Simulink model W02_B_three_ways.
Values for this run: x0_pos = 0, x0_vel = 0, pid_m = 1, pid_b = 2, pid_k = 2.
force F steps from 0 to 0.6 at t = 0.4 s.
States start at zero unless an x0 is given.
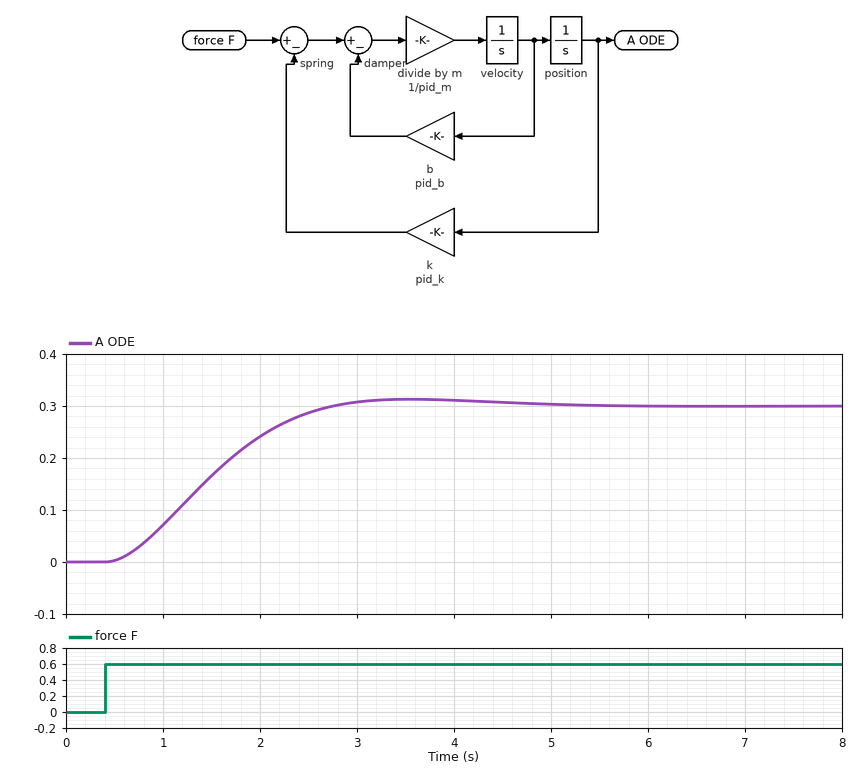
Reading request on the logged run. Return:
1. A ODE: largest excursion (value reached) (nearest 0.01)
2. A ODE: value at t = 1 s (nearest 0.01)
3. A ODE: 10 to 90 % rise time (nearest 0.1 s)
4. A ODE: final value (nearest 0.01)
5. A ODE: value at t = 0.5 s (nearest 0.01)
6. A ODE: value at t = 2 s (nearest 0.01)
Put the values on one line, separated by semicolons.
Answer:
0.31; 0.07; 1.5 s; 0.30; 0.00; 0.24
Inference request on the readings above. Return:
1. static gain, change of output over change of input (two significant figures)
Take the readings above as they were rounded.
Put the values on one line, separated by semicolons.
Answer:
0.50
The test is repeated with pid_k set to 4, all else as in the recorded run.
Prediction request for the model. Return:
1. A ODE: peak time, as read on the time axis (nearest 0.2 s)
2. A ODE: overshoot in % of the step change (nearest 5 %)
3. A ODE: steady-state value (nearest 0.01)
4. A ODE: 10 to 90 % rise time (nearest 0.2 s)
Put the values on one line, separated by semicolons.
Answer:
2.2 s; 15 %; 0.15; 0.8 s
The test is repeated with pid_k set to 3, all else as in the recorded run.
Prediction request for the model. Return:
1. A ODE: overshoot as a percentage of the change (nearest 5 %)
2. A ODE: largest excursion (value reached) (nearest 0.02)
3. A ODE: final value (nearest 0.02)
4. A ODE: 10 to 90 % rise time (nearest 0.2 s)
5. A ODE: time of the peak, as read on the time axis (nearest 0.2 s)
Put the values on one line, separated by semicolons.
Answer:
10 %; 0.22; 0.20; 1.0 s; 2.6 s
